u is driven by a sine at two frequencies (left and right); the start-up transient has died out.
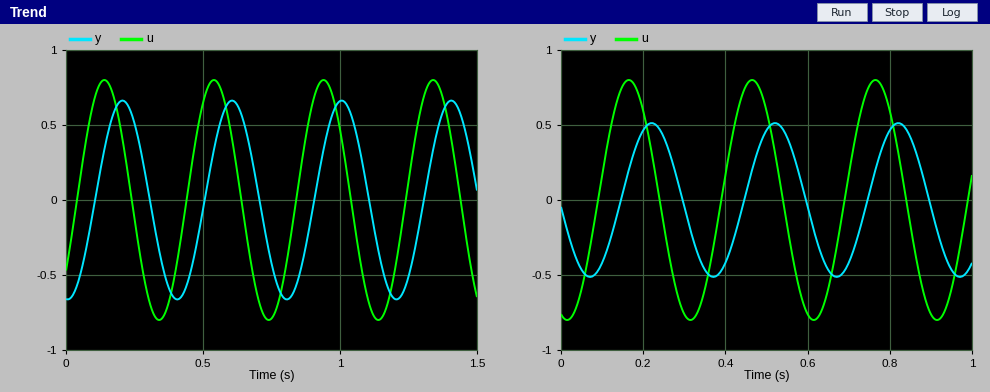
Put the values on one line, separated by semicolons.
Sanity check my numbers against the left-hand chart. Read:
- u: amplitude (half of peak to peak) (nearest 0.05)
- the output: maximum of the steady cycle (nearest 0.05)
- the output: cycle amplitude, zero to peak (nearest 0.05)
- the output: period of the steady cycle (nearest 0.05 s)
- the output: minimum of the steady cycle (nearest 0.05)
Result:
0.80; 0.65; 0.65; 0.40 s; -0.65
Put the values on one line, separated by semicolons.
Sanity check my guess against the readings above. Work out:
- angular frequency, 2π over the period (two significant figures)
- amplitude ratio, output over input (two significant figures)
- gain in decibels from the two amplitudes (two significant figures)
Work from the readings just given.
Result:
16 rad/s; 0.81; -1.8 dB
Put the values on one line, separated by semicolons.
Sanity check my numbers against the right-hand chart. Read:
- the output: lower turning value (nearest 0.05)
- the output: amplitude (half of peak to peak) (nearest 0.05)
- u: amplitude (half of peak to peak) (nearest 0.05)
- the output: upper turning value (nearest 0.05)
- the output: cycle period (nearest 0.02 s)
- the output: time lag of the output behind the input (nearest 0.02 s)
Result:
-0.50; 0.50; 0.80; 0.50; 0.30 s; 0.06 s
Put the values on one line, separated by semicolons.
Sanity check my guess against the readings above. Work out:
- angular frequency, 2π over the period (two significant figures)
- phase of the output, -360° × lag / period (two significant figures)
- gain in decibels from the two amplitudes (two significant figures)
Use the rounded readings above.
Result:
21 rad/s; -72°; -4.1 dB
